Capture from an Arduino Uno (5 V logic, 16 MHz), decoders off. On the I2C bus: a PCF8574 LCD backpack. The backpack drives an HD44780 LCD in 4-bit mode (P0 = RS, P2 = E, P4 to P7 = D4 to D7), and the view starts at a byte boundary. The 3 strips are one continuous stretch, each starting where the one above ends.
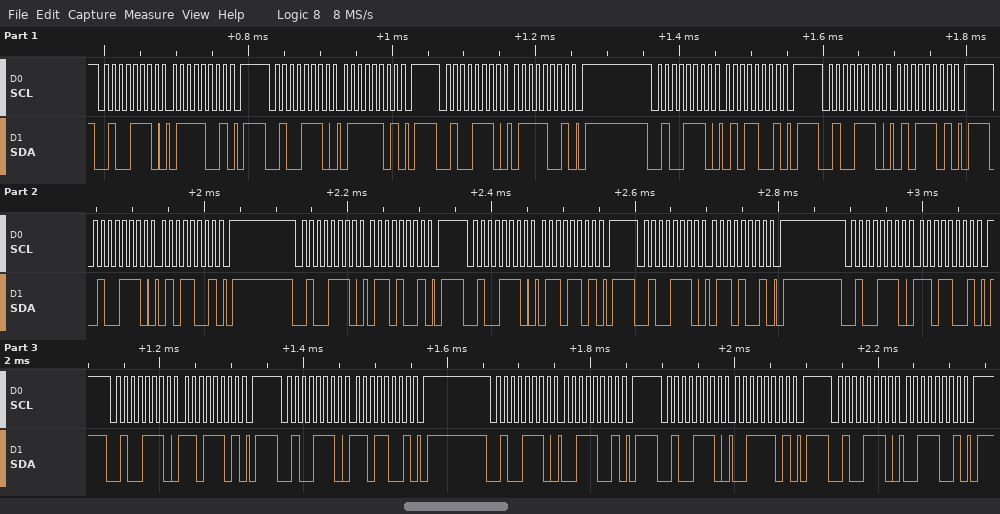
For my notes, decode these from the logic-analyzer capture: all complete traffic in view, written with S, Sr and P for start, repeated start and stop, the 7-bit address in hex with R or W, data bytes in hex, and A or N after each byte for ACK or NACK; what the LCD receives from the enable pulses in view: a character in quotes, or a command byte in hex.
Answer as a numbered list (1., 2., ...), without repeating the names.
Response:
1. S 27W A 79 A P S 27W A 7D A P S 27W A 79 A P S 27W A 59 A P S 27W A 5D A P S 27W A 59 A P S 27W A 69 A P S 27W A 6D A P S 27W A 69 A P S 27W A D9 A P S 27W A DD A P S 27W A D9 A P S 27W A 39 A P S 27W A 3D A P S 27W A 39 A P
2. 'u' 'm'
